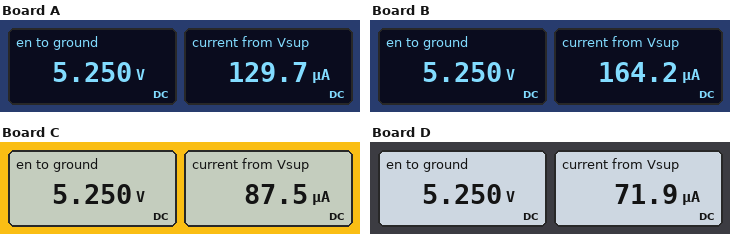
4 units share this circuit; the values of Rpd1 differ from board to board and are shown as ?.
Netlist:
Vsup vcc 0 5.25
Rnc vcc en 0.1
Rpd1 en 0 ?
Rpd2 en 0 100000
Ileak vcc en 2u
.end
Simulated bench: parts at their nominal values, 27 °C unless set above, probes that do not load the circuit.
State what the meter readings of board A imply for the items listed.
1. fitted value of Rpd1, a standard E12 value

68 kΩ
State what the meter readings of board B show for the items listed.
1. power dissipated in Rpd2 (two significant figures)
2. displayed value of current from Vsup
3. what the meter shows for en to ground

280 µW
164.2 µA
5.250 V
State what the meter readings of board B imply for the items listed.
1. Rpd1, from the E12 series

47 kΩ
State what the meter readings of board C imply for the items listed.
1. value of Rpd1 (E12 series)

150 kΩ
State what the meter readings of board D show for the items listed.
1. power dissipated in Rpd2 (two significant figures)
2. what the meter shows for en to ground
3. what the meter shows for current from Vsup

280 µW
5.250 V
71.9 µA
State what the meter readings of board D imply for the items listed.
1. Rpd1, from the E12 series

270 kΩ
